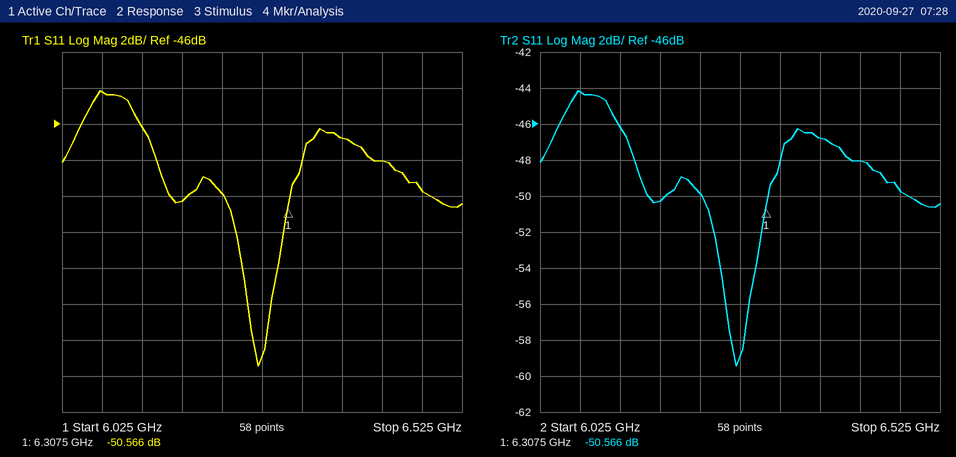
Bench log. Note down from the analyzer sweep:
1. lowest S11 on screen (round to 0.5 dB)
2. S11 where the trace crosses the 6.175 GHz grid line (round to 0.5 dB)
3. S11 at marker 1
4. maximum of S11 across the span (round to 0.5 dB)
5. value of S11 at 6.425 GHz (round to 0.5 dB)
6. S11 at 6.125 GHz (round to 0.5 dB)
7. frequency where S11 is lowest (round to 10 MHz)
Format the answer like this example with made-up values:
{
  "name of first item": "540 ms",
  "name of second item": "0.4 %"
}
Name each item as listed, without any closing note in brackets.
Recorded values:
{
  "lowest S11 on screen": "-59.5 dB",
  "S11 where the trace crosses the 6.175 GHz grid line": "-50.5 dB",
  "S11 at marker 1": "-50.566 dB",
  "maximum of S11 across the span": "-44.0 dB",
  "value of S11 at 6.425 GHz": "-48.0 dB",
  "S11 at 6.125 GHz": "-46.0 dB",
  "frequency where S11 is lowest": "6.27 GHz"
}
